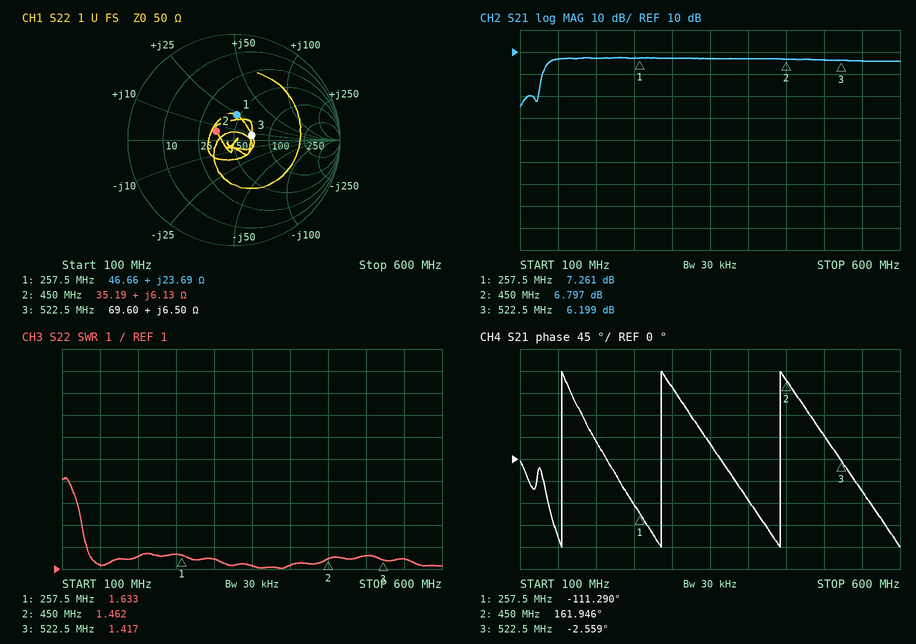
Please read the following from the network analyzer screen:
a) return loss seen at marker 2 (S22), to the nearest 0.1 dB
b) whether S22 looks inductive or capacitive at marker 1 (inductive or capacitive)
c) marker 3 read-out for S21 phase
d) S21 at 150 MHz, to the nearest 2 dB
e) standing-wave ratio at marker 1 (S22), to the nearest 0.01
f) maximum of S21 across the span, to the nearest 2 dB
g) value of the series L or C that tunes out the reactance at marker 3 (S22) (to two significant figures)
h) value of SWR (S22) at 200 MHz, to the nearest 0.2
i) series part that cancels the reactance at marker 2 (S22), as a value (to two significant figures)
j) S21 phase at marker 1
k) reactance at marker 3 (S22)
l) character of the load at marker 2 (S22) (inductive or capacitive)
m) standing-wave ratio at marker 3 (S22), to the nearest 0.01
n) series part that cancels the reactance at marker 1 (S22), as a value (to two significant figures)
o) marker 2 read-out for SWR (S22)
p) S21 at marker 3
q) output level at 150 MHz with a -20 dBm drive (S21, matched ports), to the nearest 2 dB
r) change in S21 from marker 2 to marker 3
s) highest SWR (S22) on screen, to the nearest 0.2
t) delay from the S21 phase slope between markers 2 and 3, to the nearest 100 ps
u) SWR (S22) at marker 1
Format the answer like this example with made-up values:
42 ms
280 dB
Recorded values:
14.5 dB
inductive
-2.559°
6 dB
1.63
8 dB
47 pF
1.6
58 pF
-111.290°
+6.50 Ω
inductive
1.42
26 pF
1.462
6.199 dB
-14 dBm
-0.598 dB
5.2
6.3 ns
1.633
